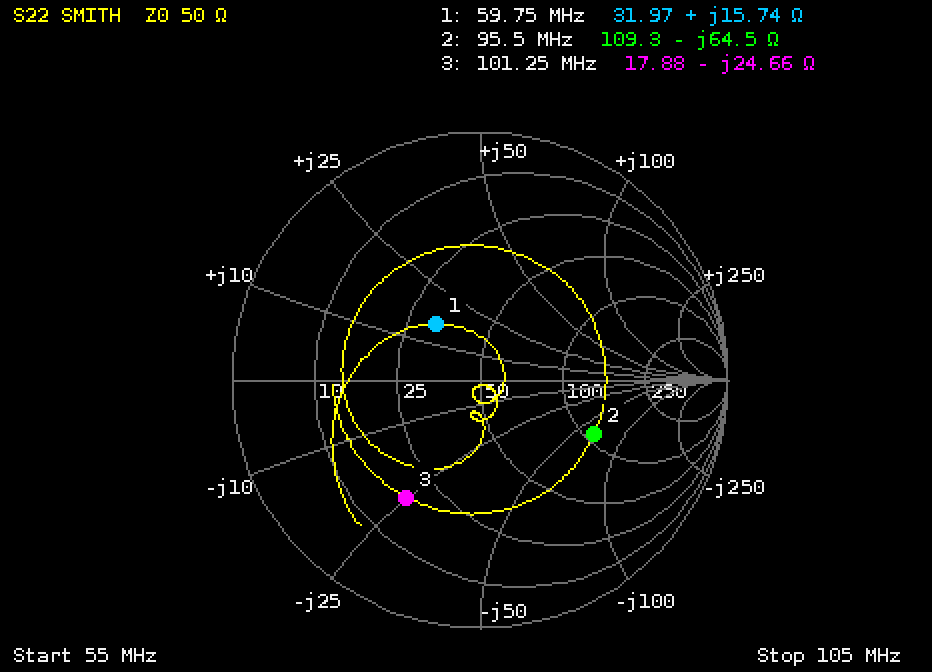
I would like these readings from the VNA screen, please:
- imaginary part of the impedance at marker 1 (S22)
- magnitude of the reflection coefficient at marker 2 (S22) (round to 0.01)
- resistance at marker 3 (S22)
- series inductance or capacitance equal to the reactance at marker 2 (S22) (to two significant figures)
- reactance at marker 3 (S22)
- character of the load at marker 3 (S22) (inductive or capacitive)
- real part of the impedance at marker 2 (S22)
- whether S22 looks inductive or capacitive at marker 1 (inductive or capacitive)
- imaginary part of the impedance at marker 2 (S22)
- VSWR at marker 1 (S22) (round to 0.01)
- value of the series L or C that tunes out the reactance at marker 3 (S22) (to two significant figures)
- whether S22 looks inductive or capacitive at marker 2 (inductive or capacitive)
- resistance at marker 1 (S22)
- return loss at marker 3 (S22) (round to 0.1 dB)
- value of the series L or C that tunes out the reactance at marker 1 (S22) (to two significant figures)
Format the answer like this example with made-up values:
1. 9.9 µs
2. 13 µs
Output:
1. +15.74 Ω
2. 0.51
3. 17.88 Ω
4. 26 pF
5. -24.66 Ω
6. capacitive
7. 109.3 Ω
8. inductive
9. -64.5 Ω
10. 1.80
11. 39 nH
12. capacitive
13. 31.97 Ω
14. 5.0 dB
15. 170 pF
